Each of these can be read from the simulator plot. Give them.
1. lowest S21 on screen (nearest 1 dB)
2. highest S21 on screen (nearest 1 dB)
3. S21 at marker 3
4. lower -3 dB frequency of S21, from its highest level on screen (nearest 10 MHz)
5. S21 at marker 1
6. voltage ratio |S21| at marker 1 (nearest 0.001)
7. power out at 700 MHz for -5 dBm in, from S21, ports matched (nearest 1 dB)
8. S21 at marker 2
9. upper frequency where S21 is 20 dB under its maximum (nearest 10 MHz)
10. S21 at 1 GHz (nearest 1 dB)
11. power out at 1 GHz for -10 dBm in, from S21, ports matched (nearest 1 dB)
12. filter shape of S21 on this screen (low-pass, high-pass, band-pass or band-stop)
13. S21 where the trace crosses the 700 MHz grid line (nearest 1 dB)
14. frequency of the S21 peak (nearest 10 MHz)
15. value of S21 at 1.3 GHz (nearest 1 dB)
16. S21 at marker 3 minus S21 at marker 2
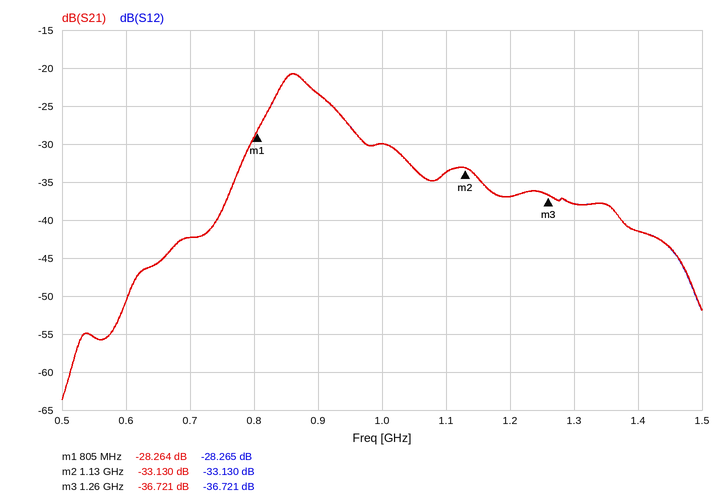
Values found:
-64 dB
-21 dB
-36.721 dB
830 MHz
-28.264 dB
0.039
-47 dBm
-33.130 dB
1.38 GHz
-30 dB
-40 dBm
band-pass
-42 dB
860 MHz
-38 dB
-3.591 dB
